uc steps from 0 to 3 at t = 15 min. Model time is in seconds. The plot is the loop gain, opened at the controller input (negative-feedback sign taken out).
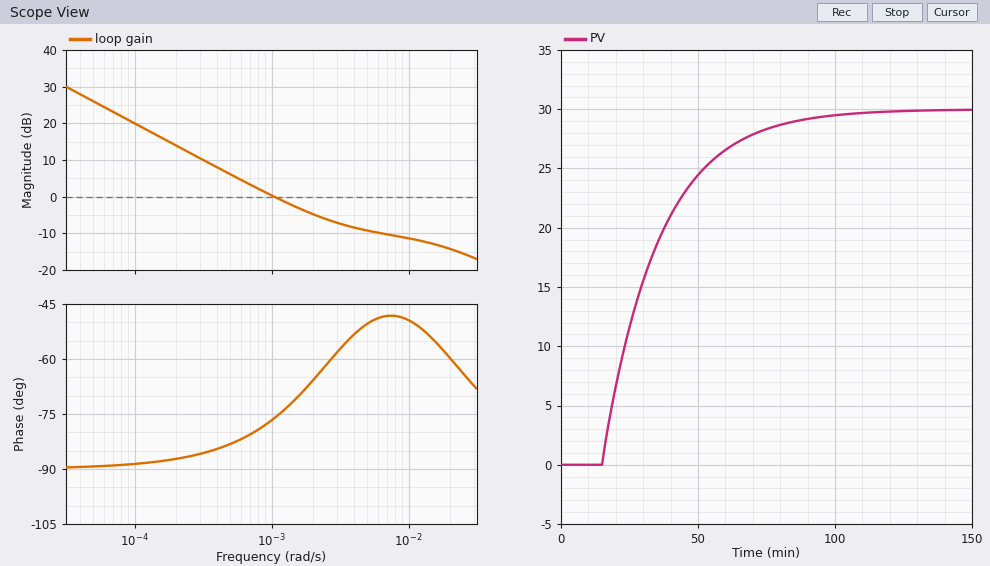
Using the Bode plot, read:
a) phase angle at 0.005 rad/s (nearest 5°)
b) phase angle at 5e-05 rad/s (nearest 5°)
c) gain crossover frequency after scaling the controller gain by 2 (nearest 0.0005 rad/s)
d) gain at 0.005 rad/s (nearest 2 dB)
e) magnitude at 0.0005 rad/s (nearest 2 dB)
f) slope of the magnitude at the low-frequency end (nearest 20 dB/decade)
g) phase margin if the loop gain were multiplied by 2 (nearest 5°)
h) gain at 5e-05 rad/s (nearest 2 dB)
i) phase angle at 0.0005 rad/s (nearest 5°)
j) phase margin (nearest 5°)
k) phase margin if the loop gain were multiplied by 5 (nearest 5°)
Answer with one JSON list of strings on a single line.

["-50°", "-90°", "0.0025 rad/s", "-10 dB", "6 dB", "-20 dB/decade", "120°", "26 dB", "-85°", "105°", "120°"]
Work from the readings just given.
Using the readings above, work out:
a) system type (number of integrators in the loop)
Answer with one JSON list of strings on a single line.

["1"]
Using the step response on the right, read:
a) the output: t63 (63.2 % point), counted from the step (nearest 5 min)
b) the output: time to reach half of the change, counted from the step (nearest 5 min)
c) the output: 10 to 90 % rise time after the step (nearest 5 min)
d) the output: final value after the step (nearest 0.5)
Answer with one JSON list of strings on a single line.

["20 min", "15 min", "45 min", "30.0"]
